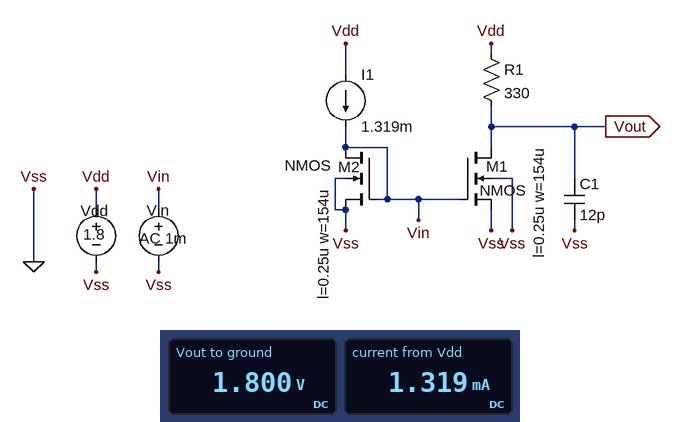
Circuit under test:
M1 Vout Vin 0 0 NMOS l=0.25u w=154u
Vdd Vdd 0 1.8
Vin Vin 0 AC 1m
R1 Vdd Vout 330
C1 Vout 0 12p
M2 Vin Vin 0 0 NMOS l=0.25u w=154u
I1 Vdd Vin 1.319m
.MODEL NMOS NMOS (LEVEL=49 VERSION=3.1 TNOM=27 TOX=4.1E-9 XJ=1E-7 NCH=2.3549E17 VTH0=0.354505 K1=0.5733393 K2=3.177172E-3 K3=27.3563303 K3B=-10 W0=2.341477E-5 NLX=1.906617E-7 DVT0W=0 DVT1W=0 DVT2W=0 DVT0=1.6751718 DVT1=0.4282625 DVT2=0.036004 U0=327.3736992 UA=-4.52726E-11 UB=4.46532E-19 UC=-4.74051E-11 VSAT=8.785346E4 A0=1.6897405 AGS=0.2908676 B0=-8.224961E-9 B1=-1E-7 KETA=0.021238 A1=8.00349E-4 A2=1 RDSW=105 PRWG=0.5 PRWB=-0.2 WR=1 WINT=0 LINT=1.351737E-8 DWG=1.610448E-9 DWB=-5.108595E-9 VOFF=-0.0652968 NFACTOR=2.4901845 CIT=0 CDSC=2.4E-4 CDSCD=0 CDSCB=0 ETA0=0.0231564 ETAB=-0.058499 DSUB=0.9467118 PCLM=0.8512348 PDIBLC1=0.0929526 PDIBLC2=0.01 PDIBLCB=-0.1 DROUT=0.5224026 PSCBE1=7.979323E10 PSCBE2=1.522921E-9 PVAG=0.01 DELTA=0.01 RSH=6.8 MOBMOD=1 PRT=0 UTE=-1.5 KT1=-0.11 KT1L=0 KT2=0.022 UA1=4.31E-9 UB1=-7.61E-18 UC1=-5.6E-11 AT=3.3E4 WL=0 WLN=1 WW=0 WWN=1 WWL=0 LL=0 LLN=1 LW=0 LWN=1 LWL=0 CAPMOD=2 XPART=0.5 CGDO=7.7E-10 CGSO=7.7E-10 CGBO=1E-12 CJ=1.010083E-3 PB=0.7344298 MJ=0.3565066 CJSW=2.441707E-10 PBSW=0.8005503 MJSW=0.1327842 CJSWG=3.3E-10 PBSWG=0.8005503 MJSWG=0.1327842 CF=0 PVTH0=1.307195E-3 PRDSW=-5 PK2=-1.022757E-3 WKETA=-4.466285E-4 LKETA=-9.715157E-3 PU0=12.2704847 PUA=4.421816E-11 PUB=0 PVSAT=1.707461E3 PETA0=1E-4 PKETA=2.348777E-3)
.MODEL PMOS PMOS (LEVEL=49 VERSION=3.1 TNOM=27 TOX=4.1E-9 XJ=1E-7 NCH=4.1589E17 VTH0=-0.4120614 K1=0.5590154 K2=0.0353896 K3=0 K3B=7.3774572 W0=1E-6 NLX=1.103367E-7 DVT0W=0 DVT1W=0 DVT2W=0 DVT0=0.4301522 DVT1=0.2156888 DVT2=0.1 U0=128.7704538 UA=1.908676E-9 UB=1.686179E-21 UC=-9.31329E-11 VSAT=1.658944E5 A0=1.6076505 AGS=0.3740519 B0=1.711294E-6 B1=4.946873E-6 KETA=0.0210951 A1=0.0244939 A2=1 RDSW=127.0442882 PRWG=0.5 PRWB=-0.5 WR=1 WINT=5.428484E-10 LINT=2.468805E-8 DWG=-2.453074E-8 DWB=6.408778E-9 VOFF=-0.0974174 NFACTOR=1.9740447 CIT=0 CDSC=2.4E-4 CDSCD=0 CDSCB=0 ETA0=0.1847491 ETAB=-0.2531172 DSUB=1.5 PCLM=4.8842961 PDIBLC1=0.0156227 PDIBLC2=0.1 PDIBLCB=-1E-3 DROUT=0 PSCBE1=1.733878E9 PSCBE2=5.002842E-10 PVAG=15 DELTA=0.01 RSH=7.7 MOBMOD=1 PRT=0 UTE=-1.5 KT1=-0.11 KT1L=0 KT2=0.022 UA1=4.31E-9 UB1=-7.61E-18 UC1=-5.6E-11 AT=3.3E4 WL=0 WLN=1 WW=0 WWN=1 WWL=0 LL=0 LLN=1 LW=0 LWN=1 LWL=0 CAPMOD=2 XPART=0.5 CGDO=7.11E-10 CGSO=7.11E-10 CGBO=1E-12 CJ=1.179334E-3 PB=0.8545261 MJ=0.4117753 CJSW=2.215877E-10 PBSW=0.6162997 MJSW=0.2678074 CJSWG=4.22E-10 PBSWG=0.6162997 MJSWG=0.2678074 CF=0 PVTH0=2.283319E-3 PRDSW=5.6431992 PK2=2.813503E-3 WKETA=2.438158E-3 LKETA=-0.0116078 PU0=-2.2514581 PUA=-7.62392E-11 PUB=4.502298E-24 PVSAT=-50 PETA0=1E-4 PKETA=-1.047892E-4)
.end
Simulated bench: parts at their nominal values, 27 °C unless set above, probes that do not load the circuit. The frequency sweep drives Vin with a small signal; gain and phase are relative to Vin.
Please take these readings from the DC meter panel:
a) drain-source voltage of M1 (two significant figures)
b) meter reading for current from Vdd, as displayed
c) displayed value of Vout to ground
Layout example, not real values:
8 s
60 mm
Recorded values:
1.8 V
1.319 mA
1.800 V
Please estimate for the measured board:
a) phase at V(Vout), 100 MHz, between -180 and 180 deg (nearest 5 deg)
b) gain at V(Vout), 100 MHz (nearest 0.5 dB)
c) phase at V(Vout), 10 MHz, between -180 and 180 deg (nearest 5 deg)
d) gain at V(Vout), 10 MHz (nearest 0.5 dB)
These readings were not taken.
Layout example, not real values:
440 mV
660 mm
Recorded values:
20 deg
-41.0 dB
75 deg
-52.5 dB
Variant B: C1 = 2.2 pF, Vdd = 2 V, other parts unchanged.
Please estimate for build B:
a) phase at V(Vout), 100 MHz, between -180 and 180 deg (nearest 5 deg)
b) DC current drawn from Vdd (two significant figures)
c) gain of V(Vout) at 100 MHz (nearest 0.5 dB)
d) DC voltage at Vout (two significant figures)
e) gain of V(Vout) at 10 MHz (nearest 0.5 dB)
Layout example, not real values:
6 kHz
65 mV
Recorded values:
65 deg
1.3 mA
-33.0 dB
2.0 V
-52.0 dB
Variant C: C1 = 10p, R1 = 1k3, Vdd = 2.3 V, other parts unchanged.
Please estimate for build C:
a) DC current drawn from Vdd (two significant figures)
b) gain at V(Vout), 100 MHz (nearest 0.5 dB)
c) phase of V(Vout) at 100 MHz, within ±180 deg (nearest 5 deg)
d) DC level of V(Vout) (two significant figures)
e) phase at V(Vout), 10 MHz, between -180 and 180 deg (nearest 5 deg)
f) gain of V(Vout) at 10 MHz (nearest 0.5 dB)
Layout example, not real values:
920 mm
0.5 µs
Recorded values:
1.3 mA
-38.5 dB
5 deg
2.3 V
50 deg
-42.5 dB
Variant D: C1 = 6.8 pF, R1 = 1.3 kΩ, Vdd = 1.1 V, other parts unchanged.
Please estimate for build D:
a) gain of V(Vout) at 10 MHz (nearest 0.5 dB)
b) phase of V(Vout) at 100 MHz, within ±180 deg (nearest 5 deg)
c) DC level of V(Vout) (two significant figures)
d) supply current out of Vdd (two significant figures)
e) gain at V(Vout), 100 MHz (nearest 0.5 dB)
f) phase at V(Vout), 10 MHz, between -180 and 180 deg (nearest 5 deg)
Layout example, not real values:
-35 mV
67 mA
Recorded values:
-41.5 dB
10 deg
1.1 V
1.3 mA
-35.5 dB
60 deg
